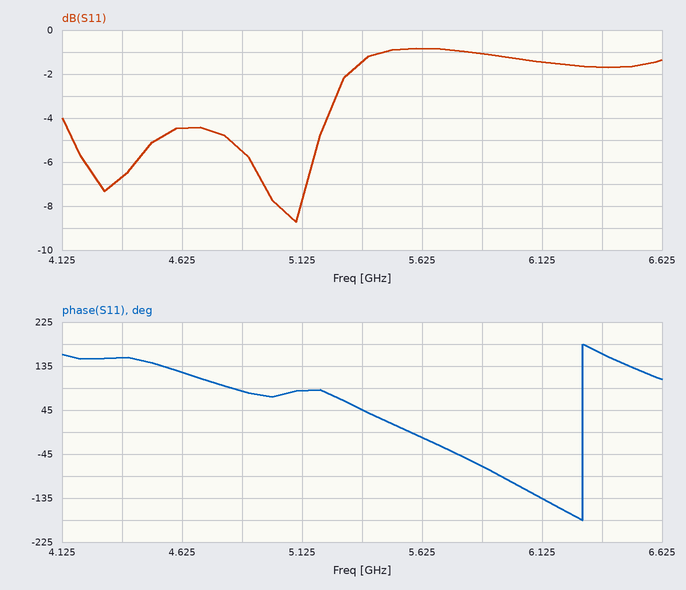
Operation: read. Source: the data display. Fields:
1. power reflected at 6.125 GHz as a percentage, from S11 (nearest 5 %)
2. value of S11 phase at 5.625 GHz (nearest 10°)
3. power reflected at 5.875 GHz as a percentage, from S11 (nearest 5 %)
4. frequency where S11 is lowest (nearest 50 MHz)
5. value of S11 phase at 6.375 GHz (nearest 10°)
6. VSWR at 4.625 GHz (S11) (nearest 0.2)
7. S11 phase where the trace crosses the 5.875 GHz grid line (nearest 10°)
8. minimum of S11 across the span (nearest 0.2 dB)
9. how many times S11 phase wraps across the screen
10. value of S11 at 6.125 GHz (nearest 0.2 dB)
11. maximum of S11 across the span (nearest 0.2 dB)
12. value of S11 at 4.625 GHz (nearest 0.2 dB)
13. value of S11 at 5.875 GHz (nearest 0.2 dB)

70 %
-10°
80 %
5.10 GHz
160°
4.0
-70°
-8.8 dB
1
-1.4 dB
-0.8 dB
-4.4 dB
-1.0 dB
